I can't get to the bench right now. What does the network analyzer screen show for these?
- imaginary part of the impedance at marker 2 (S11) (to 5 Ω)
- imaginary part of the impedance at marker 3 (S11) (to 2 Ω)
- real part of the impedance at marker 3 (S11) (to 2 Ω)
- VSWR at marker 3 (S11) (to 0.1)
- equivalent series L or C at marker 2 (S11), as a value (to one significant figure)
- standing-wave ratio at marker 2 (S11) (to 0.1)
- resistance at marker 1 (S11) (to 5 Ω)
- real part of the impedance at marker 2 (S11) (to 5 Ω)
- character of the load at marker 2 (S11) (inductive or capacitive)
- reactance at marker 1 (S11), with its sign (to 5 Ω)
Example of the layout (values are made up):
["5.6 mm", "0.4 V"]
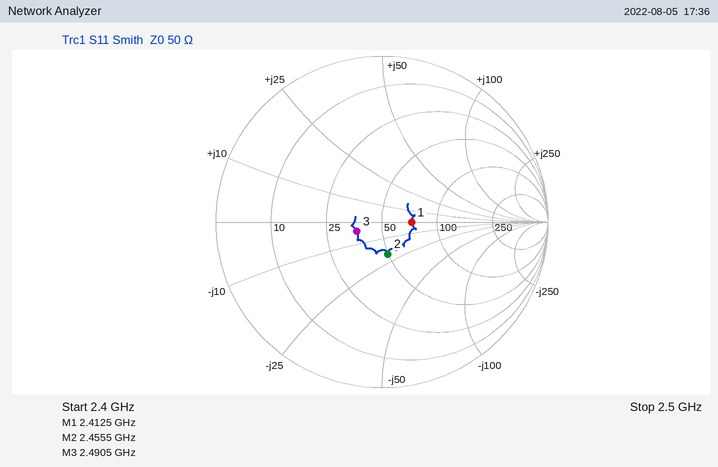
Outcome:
["-20 Ω", "-4 Ω", "36 Ω", "1.4", "3 pF", "1.5", "70 Ω", "50 Ω", "capacitive", "0 Ω"]
